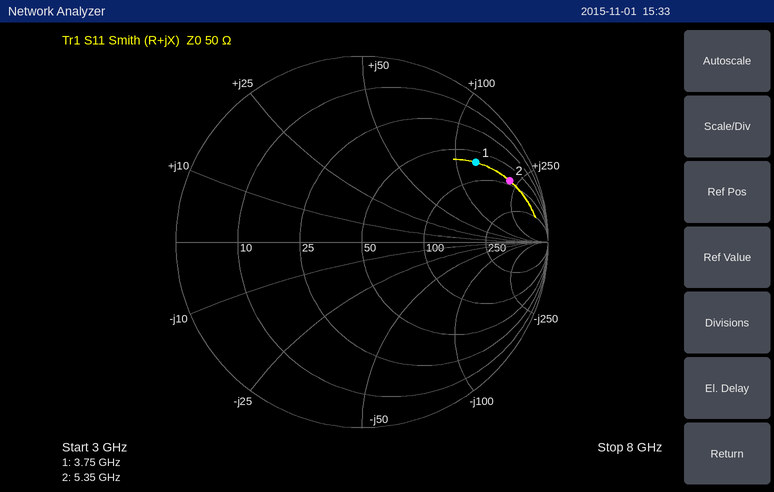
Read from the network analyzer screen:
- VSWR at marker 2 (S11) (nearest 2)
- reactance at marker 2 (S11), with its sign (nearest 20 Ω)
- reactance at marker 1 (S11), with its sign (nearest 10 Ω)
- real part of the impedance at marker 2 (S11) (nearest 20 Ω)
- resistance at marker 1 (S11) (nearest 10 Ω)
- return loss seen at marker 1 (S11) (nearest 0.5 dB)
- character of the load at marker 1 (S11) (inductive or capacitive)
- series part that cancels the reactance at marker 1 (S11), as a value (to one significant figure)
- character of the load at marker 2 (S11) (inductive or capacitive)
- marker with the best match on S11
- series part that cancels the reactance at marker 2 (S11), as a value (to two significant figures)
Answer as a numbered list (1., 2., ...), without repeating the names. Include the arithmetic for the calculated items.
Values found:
1. 14
2. +220 Ω
3. +130 Ω
4. 80 Ω
5. 70 Ω
6. 2.5 dB
7. inductive
8. C = 1/(2π × 3.75 GHz × 130 Ω) ≈ 326 fF, so 300 fF to one significant figure
9. inductive
10. marker 1
11. C = 1/(2π × 5.35 GHz × 220 Ω) ≈ 135 fF, so 140 fF to two significant figures
